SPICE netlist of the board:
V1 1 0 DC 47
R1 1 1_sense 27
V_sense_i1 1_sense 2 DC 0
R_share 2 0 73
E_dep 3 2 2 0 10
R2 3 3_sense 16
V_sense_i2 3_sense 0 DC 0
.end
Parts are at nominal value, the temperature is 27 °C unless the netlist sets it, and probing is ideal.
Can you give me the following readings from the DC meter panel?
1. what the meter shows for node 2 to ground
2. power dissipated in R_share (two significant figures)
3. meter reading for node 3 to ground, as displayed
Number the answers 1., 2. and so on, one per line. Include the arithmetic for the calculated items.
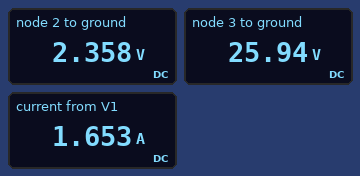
1. 2.358 V
2. (2.358 V)^2 / 73 Ω = 76 mW
3. 25.94 V
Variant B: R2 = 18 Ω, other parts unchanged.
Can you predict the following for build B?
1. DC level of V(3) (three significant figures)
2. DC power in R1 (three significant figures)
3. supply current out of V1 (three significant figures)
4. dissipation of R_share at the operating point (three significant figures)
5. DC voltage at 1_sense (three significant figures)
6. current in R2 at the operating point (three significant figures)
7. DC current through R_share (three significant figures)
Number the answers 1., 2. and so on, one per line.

1. 28.9 V
2. 72.9 W
3. 1.64 A
4. 94.8 mW
5. 2.63 V
6. 1.61 A
7. 36.0 mA
